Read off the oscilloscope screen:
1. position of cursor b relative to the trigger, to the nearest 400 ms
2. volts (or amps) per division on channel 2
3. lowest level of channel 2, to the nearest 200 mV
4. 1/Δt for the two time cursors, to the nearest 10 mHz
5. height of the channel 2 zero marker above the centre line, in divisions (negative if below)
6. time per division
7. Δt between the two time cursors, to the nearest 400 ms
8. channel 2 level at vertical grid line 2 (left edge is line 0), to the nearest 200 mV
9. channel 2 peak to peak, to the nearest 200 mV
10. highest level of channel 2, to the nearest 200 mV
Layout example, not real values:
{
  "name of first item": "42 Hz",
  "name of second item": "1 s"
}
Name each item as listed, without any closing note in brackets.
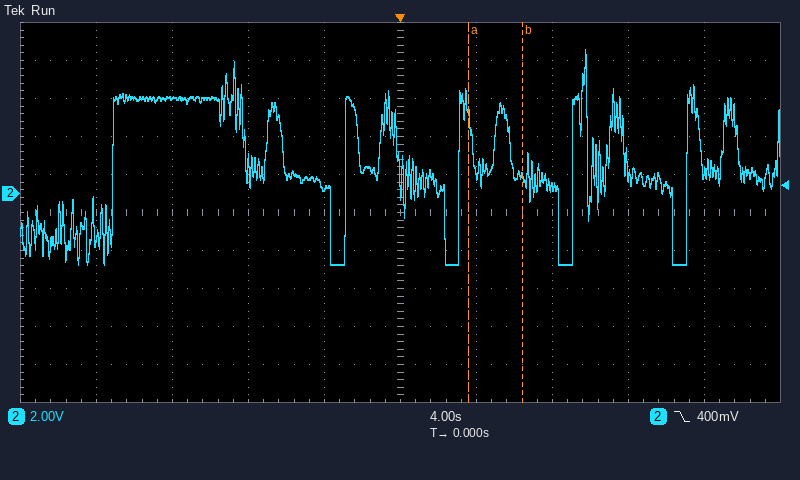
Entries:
{
  "position of cursor b relative to the trigger, to the nearest 400 ms": "+6.4 s",
  "volts (or amps) per division on channel 2": "2 V",
  "lowest level of channel 2, to the nearest 200 mV": "-3.8 V",
  "1/Δt for the two time cursors, to the nearest 10 mHz": "360 mHz",
  "height of the channel 2 zero marker above the centre line, in divisions": "+0.5 div",
  "time per division": "4 s",
  "Δt between the two time cursors, to the nearest 400 ms": "2.8 s",
  "channel 2 level at vertical grid line 2 (left edge is line 0), to the nearest 200 mV": "5.0 V",
  "channel 2 peak to peak, to the nearest 200 mV": "11.4 V",
  "highest level of channel 2, to the nearest 200 mV": "7.6 V"
}
